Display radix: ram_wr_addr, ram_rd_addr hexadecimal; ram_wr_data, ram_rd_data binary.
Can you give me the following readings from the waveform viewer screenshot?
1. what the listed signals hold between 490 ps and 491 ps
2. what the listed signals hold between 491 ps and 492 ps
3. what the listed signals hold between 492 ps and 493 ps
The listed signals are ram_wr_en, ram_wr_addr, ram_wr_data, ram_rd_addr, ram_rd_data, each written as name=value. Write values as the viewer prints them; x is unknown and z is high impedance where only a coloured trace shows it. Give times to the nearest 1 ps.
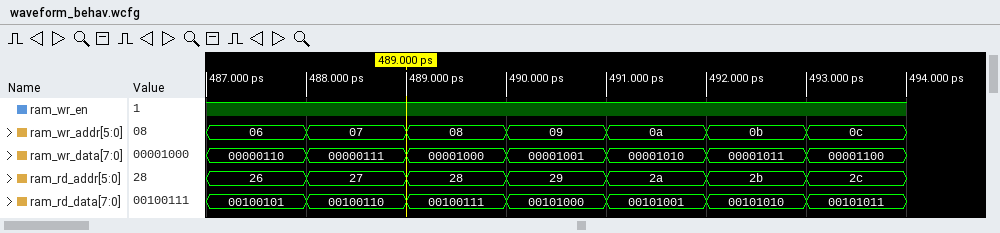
ram_wr_en=1, ram_wr_addr=09, ram_wr_data=00001001, ram_rd_addr=29, ram_rd_data=00101000
ram_wr_en=1, ram_wr_addr=0a, ram_wr_data=00001010, ram_rd_addr=2a, ram_rd_data=00101001
ram_wr_en=1, ram_wr_addr=0b, ram_wr_data=00001011, ram_rd_addr=2b, ram_rd_data=00101010
